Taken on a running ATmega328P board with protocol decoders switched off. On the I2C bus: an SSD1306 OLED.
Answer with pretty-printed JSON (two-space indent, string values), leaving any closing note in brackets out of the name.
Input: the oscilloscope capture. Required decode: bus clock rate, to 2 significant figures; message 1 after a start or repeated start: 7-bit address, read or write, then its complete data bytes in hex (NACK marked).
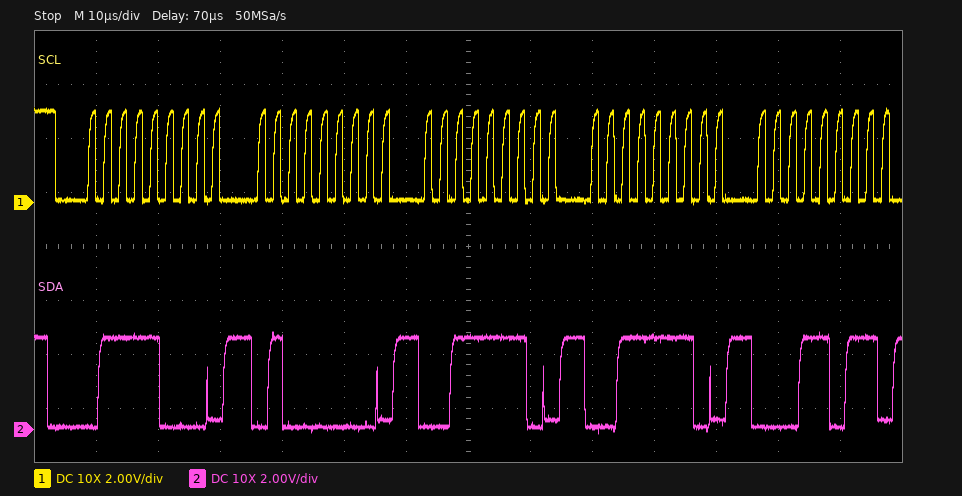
{
  "bus clock rate, to 2 significant figures": "400 kHz",
  "message 1 after a start or repeated start: 7-bit address, read or write, then its complete data bytes in hex": "0x3C write: 40 3E 3E 1B"
}
